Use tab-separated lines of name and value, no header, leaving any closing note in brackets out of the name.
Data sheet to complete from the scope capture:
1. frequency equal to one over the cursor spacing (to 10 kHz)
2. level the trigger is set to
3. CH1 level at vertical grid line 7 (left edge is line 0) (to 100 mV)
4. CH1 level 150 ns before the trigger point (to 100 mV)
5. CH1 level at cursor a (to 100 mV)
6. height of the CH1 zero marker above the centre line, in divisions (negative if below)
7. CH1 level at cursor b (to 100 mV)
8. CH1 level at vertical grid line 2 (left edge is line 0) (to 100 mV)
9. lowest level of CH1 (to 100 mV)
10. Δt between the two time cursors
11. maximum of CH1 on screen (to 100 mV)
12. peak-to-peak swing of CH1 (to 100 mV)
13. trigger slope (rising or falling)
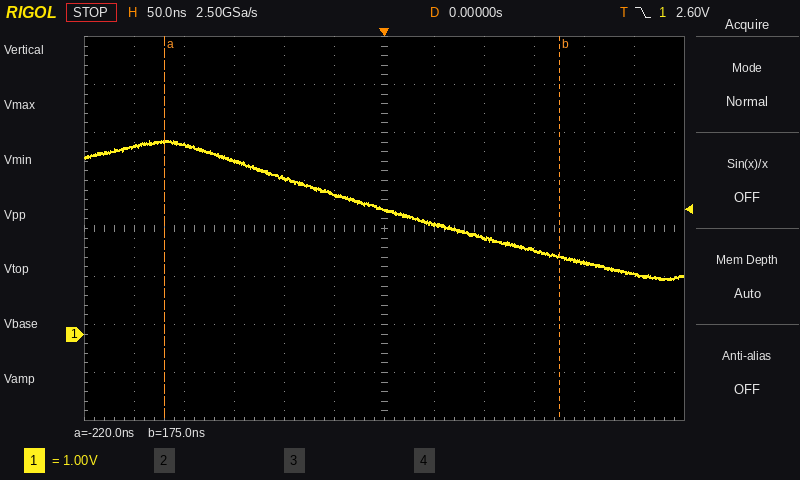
frequency equal to one over the cursor spacing	2.53 MHz
level the trigger is set to	2.60 V
CH1 level at vertical grid line 7 (left edge is line 0)	2.3 V
CH1 level 150 ns before the trigger point	3.6 V
CH1 level at cursor a	4.0 V
height of the CH1 zero marker above the centre line, in divisions	-2.2 div
CH1 level at cursor b	1.6 V
CH1 level at vertical grid line 2 (left edge is line 0)	3.9 V
lowest level of CH1	1.1 V
Δt between the two time cursors	395 ns
maximum of CH1 on screen	4.0 V
peak-to-peak swing of CH1	2.9 V
trigger slope	falling
